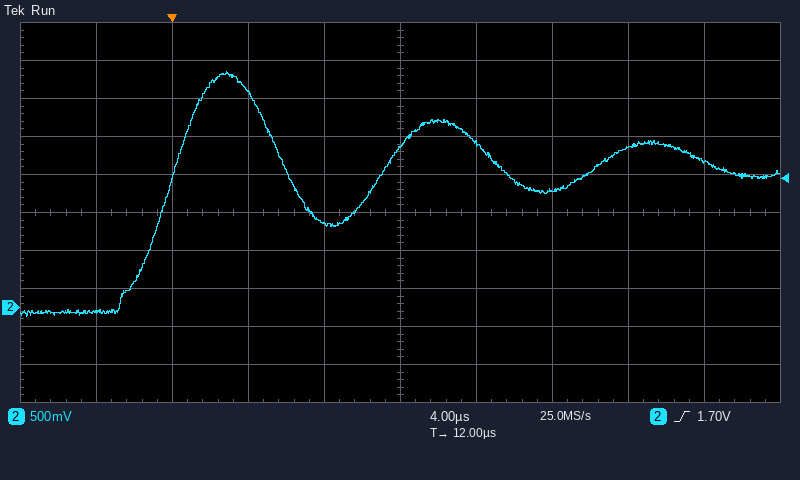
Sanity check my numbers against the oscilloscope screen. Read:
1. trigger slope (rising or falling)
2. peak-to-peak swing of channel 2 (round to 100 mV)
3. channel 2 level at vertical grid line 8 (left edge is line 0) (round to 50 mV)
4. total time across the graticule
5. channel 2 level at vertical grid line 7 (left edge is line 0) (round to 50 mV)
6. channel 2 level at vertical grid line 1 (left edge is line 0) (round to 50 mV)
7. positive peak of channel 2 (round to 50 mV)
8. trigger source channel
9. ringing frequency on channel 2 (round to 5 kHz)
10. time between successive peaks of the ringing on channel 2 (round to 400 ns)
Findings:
rising
3.20 V
2.10 V
40 µs
1.55 V
-50 mV
3.10 V
channel 2
90 kHz
11.2 µs
